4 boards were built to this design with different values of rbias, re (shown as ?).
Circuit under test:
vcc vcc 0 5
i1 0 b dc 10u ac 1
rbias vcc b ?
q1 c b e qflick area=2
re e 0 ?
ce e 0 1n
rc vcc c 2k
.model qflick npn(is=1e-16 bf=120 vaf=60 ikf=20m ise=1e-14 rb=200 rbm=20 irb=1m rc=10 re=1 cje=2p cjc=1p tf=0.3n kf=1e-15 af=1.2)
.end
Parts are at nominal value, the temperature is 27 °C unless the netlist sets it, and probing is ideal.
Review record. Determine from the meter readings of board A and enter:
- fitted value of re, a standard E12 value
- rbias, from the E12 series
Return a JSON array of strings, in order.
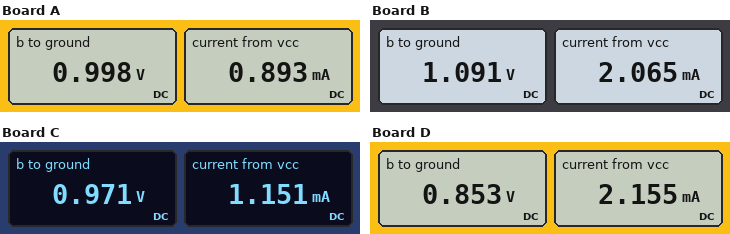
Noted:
["270 Ω", "1.5 MΩ"]
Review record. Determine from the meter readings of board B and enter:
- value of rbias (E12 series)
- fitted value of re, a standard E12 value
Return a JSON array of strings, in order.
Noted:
["220 kΩ", "150 Ω"]
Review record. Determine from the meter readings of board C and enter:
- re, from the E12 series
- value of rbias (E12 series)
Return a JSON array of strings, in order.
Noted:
["180 Ω", "680 kΩ"]
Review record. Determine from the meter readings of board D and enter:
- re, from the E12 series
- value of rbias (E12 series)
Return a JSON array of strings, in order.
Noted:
["33 Ω", "220 kΩ"]
